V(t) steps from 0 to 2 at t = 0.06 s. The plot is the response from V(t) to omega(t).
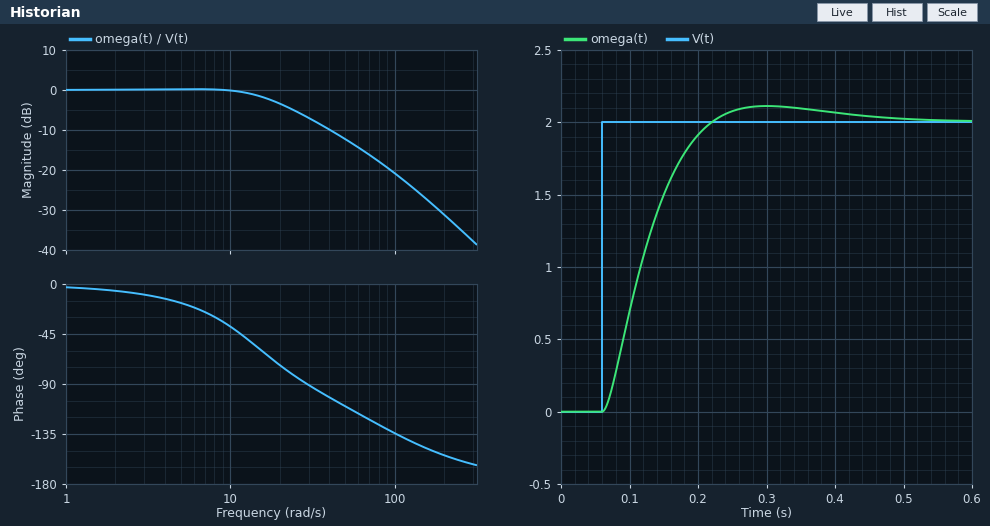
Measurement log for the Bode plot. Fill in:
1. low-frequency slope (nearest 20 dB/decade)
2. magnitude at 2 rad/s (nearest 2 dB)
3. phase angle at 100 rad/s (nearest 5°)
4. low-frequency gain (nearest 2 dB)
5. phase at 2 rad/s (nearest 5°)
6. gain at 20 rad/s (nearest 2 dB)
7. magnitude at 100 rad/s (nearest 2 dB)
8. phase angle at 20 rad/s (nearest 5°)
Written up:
0 dB/decade
0 dB
-135°
0 dB
-5°
-4 dB
-20 dB
-75°
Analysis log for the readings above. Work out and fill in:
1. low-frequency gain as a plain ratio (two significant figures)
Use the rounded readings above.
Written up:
1.0
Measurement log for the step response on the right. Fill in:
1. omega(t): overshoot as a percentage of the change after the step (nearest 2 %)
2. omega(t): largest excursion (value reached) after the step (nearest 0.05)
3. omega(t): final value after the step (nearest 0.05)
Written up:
6 %
2.10
2.00
